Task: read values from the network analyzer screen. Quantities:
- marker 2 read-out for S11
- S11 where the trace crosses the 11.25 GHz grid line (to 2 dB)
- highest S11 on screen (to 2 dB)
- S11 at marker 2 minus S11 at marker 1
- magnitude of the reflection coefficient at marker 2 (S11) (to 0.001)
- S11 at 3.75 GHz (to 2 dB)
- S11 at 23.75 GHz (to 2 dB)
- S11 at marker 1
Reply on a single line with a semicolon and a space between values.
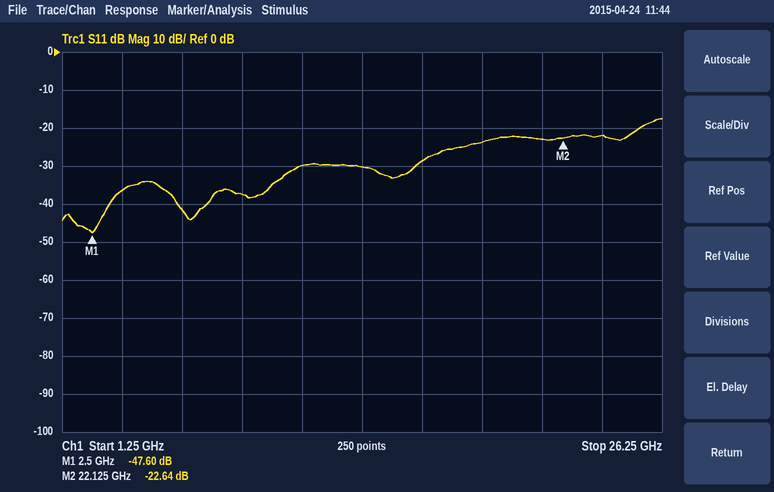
-22.64 dB; -30 dB; -18 dB; 24.96 dB; 0.074; -36 dB; -22 dB; -47.60 dB
